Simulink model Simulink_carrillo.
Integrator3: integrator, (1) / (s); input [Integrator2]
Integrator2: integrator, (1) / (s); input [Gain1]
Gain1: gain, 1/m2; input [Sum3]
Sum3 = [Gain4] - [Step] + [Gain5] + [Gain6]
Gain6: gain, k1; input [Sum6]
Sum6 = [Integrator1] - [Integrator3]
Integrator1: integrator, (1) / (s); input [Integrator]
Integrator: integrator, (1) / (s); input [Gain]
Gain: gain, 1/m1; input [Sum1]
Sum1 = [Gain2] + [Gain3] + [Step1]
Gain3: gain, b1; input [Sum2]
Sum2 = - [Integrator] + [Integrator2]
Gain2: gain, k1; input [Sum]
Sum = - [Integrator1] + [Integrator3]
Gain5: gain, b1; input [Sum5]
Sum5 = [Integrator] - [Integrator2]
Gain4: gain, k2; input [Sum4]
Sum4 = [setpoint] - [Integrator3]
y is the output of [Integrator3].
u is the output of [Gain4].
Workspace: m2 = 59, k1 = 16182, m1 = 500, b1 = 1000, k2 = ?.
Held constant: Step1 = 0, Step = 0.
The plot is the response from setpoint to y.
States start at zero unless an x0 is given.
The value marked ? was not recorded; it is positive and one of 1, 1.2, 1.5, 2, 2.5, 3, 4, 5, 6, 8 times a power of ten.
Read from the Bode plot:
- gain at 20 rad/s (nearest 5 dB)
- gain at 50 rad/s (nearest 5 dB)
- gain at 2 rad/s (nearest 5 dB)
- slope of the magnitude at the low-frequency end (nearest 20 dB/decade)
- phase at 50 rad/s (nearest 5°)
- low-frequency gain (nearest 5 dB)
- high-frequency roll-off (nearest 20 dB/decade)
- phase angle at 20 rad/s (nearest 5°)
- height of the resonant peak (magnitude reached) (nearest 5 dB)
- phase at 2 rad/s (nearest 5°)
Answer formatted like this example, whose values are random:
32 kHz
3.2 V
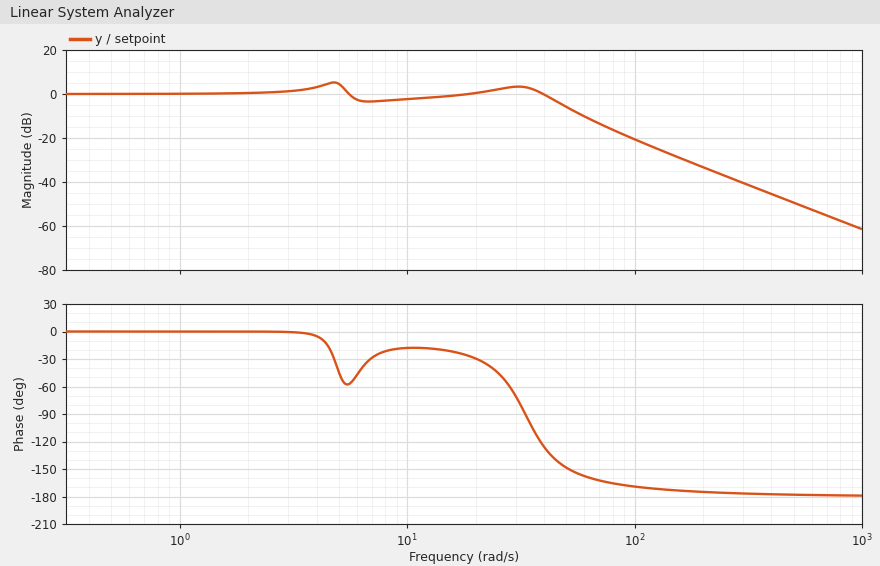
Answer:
0 dB
-5 dB
0 dB
0 dB/decade
-150°
0 dB
-40 dB/decade
-30°
5 dB
0°
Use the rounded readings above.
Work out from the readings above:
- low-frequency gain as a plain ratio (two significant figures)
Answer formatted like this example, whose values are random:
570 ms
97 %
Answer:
1.0
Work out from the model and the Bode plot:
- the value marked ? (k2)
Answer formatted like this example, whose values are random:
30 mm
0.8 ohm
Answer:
50000
